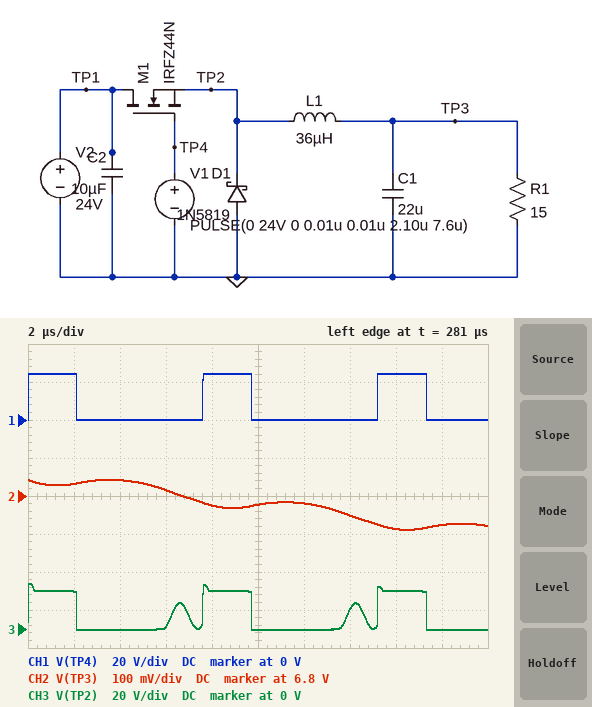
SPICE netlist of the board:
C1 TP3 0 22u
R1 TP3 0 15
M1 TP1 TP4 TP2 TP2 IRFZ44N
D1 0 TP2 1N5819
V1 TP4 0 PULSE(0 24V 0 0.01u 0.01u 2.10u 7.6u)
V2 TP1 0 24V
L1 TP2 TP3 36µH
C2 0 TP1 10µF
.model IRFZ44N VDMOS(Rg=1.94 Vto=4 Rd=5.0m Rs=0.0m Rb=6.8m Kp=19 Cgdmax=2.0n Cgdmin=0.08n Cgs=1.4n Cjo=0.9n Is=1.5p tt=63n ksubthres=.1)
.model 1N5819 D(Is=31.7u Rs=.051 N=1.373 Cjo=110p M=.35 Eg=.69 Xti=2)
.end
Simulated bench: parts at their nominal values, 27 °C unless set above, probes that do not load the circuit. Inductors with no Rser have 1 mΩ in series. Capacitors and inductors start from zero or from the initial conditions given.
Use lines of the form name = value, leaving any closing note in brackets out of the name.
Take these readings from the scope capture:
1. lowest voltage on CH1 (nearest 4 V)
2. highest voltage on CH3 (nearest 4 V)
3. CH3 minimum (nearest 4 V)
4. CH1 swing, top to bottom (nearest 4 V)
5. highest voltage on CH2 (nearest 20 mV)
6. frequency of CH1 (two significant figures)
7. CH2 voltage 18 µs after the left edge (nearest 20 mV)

lowest voltage on CH1 = 0 V
highest voltage on CH3 = 24 V
CH3 minimum = 0 V
CH1 swing, top to bottom = 24 V
highest voltage on CH2 = 6.84 V
frequency of CH1 = 130 kHz
CH2 voltage 18 µs after the left edge = 6.72 V
